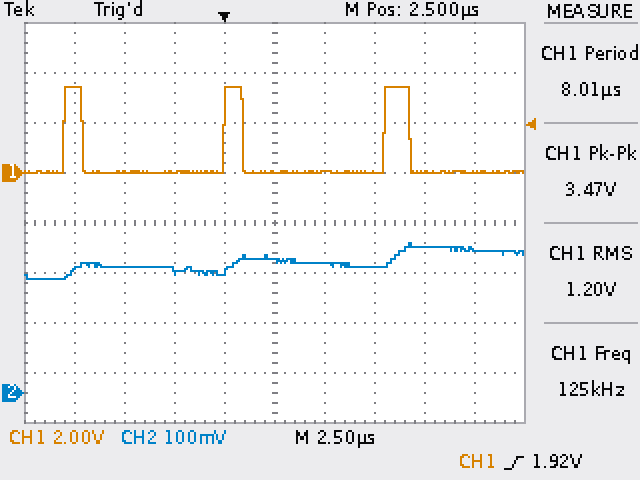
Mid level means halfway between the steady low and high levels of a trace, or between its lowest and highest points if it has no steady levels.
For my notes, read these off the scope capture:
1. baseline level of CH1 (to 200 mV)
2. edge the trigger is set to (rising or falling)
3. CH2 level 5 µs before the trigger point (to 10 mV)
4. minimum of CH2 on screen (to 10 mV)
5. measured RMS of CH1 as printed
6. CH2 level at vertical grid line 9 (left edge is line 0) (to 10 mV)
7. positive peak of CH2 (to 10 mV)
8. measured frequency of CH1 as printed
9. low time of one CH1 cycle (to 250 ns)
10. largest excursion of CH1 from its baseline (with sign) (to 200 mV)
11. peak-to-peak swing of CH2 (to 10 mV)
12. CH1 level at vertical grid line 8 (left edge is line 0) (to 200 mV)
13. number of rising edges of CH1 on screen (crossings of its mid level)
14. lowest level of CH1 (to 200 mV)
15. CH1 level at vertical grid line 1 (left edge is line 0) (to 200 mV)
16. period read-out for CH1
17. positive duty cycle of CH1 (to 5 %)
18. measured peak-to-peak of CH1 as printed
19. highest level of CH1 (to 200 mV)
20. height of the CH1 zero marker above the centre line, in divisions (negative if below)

0.0 V
rising
250 mV
230 mV
1.20 V
290 mV
300 mV
125 kHz
7.00 µs
+3.4 V
70 mV
0.0 V
3
0.0 V
3.4 V
8.01 µs
15 %
3.47 V
3.4 V
+1.0 div
